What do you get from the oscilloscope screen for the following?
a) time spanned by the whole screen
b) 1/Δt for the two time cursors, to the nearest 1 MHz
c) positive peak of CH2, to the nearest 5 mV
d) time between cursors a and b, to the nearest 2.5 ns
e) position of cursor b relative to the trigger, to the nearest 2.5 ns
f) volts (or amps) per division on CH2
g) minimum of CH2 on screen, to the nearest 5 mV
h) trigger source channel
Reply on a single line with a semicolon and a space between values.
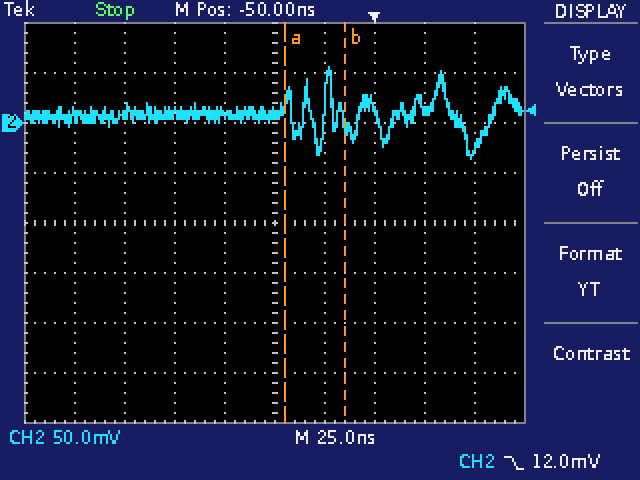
250 ns; 33 MHz; 55 mV; 30.0 ns; -15.0 ns; 50 mV; -35 mV; CH2
